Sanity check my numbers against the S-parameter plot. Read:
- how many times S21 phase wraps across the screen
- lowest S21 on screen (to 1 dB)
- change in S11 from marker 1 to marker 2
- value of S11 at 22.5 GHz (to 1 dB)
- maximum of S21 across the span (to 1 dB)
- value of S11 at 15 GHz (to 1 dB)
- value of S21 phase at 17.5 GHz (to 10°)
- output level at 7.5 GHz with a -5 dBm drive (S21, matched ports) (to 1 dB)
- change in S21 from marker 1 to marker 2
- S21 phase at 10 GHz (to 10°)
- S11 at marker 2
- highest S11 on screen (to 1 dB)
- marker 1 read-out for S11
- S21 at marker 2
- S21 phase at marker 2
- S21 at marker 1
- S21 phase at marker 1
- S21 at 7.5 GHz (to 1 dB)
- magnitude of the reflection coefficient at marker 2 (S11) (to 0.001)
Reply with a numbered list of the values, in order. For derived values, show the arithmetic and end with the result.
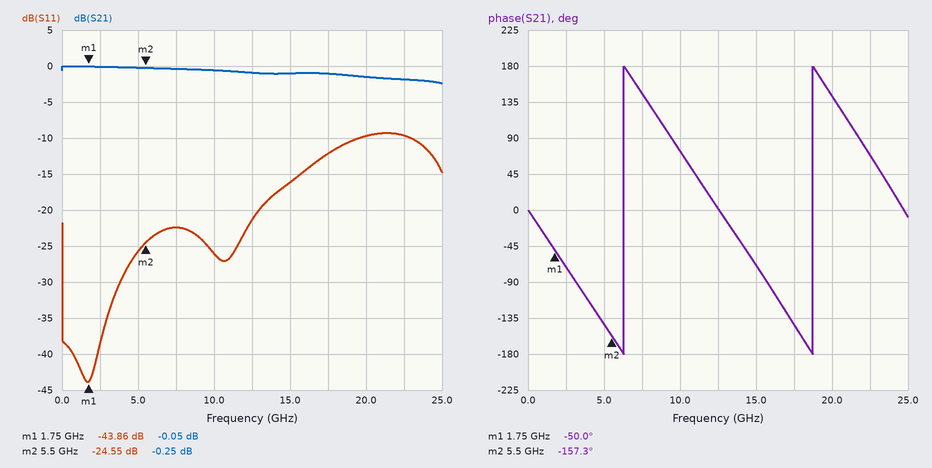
1. 2
2. -2 dB
3. -24.55 − (-43.86) = 19.31 dB
4. -10 dB
5. 0 dB
6. -16 dB
7. -140°
8. -5 dBm + (0 dB) = -5 dBm
9. -0.25 − (-0.05) = -0.20 dB
10. 70°
11. -24.55 dB
12. -9 dB
13. -43.86 dB
14. -0.25 dB
15. -157.3°
16. -0.05 dB
17. -50.0°
18. 0 dB
19. 10^(-24.55/20) ≈ 0.059
